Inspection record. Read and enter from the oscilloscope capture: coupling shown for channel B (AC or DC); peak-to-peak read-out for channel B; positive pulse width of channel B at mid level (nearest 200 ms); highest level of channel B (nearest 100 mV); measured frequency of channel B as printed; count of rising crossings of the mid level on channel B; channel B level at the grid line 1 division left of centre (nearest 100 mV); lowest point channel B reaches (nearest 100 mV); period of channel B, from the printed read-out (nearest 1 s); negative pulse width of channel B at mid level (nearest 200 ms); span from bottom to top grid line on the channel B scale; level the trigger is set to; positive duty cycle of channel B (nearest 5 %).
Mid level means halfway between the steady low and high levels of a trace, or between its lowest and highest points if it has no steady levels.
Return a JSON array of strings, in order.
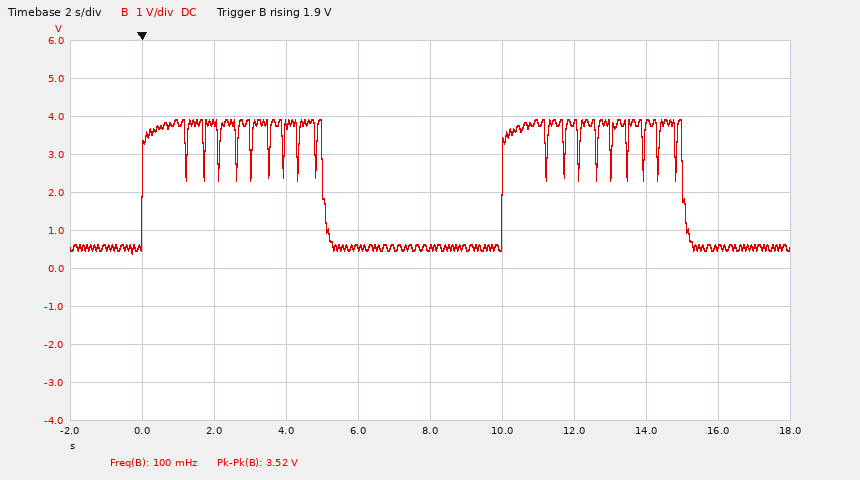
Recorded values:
["DC", "3.52 V", "5.0 s", "3.9 V", "100 mHz", "2", "600 mV", "400 mV", "10 s", "5.0 s", "10 V", "1.9 V", "50 %"]
